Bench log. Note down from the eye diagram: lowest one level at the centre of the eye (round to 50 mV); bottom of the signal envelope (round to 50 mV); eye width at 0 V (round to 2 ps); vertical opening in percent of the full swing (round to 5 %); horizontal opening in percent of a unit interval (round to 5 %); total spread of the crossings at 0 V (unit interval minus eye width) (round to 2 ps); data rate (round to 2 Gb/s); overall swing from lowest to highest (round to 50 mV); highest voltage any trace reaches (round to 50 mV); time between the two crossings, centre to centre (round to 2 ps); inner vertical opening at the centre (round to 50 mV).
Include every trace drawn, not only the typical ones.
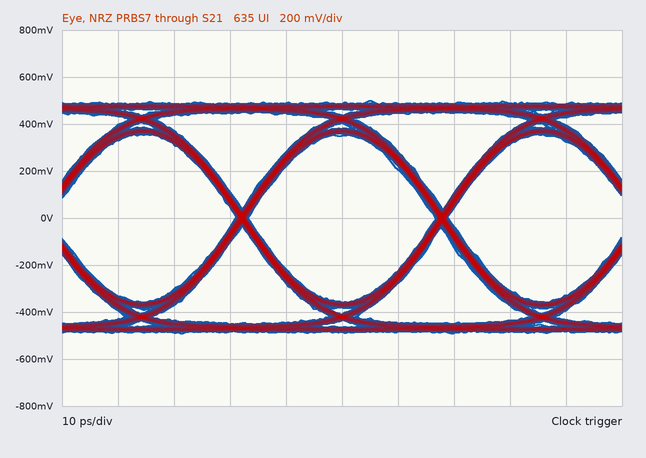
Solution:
350 mV
-500 mV
34 ps
70 %
95 %
2 ps
28 Gb/s
1.00 V
500 mV
36 ps
700 mV
